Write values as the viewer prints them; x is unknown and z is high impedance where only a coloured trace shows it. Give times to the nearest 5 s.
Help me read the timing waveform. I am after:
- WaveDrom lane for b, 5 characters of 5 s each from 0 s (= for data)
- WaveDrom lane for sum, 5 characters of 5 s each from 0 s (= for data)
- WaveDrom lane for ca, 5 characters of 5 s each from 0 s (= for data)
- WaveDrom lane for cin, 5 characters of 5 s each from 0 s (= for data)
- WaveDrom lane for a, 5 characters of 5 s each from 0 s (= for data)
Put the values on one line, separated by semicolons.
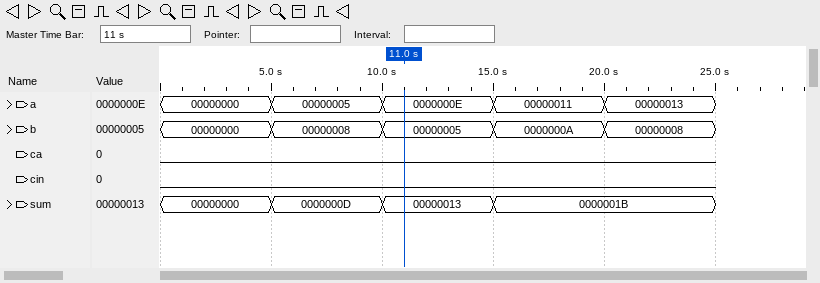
{name: 'b', wave: '=====', data: '00000000 00000008 00000005 0000000A 00000008'}; {name: 'sum', wave: '====.', data: '00000000 0000000D 00000013 0000001B'}; {name: 'ca', wave: '0....'}; {name: 'cin', wave: '0....'}; {name: 'a', wave: '=====', data: '00000000 00000005 0000000E 00000011 00000013'}
